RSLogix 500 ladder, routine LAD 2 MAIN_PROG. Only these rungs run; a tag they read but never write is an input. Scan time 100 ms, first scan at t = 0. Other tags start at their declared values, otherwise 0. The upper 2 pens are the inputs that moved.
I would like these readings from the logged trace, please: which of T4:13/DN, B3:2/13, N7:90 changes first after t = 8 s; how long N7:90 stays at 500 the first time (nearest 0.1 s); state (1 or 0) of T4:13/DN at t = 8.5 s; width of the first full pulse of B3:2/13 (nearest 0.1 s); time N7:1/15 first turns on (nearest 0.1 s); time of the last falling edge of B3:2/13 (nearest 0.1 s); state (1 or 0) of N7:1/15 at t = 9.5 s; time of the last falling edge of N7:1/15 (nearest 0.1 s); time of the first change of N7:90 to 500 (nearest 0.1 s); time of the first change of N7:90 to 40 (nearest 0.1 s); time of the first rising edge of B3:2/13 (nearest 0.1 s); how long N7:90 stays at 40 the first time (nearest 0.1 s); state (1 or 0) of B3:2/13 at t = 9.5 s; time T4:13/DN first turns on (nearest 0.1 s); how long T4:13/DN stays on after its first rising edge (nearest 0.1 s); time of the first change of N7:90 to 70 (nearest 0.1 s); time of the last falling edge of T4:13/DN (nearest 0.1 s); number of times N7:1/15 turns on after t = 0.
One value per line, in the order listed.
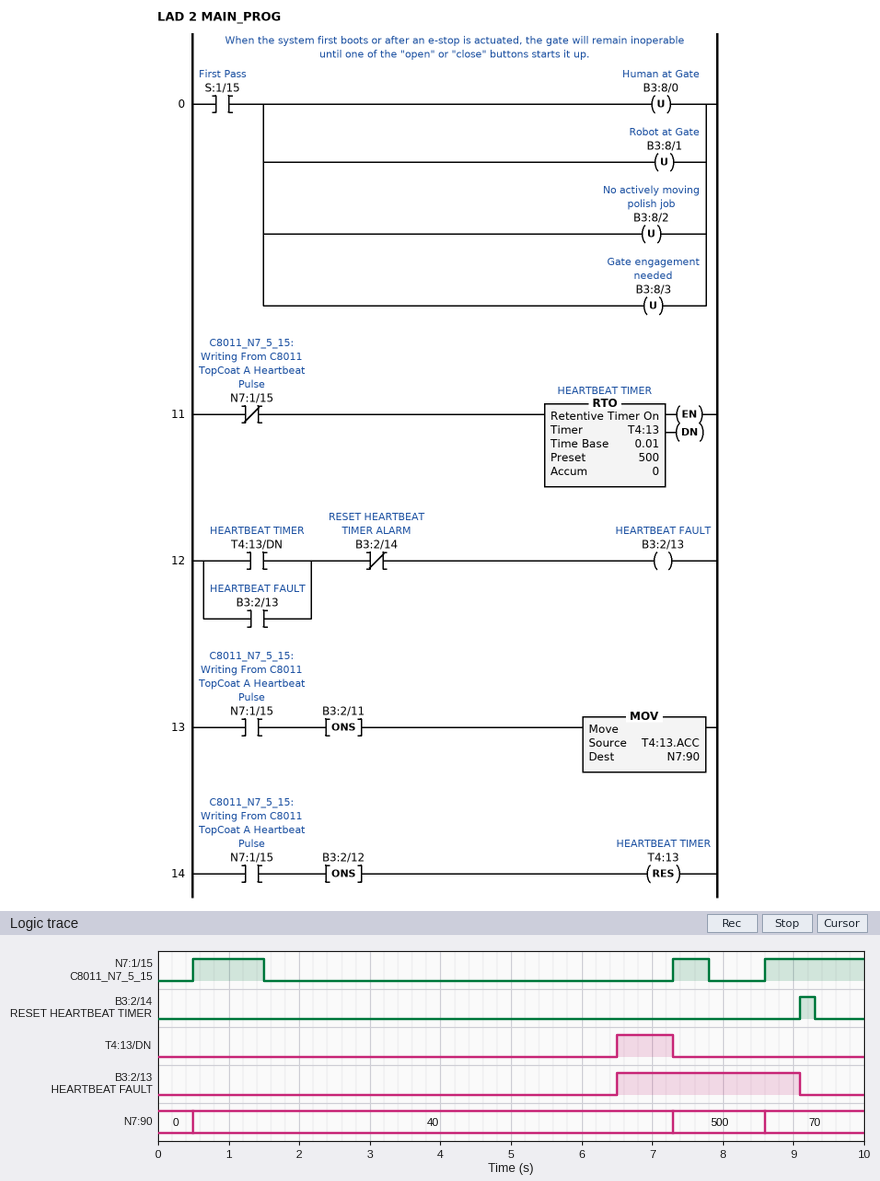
N7:90
1.3 s
0
2.6 s
0.5 s
9.1 s
1
7.8 s
7.3 s
0.5 s
6.5 s
6.8 s
0
6.5 s
0.8 s
8.6 s
7.3 s
3
